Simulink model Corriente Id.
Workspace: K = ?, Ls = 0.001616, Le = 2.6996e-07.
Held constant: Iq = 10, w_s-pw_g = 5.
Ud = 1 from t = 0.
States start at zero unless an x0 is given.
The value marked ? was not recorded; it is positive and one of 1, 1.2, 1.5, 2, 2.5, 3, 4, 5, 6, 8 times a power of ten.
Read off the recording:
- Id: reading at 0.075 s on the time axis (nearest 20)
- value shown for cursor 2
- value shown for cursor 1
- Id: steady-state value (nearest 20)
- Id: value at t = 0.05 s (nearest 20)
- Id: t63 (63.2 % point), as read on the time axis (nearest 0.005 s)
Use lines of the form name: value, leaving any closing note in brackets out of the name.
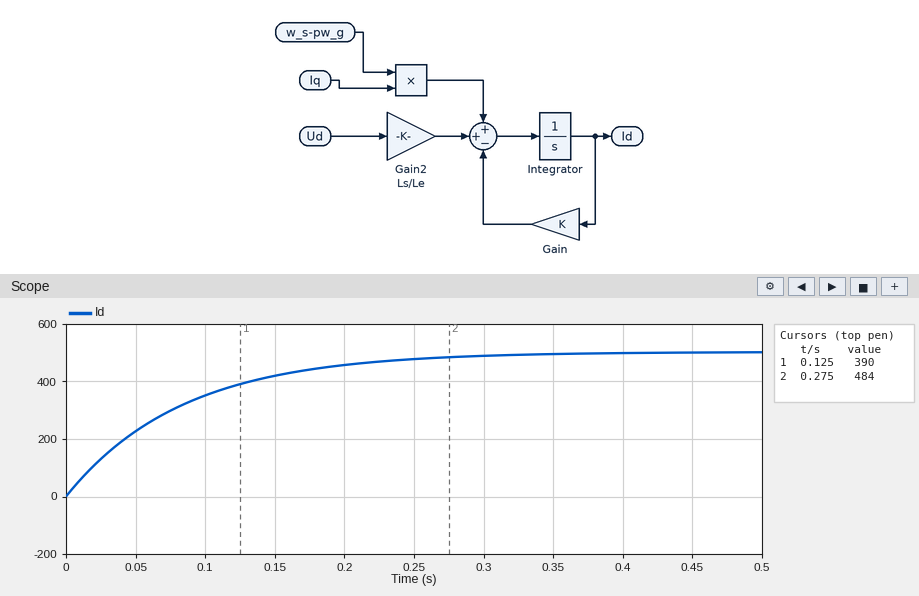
Id: reading at 0.075 s on the time axis: 300
value shown for cursor 2: 484
value shown for cursor 1: 390
Id: steady-state value: 500
Id: value at t = 0.05 s: 220
Id: t63 (63.2 % point), as read on the time axis: 0.085 s
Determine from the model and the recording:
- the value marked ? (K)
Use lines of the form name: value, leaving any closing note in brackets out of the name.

the value marked ?: 12
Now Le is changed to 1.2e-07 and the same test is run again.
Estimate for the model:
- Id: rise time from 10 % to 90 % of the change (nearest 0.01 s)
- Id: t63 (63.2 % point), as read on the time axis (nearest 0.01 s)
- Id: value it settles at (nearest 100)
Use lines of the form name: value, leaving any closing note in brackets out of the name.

Id: rise time from 10 % to 90 % of the change: 0.18 s
Id: t63 (63.2 % point), as read on the time axis: 0.08 s
Id: value it settles at: 1100
